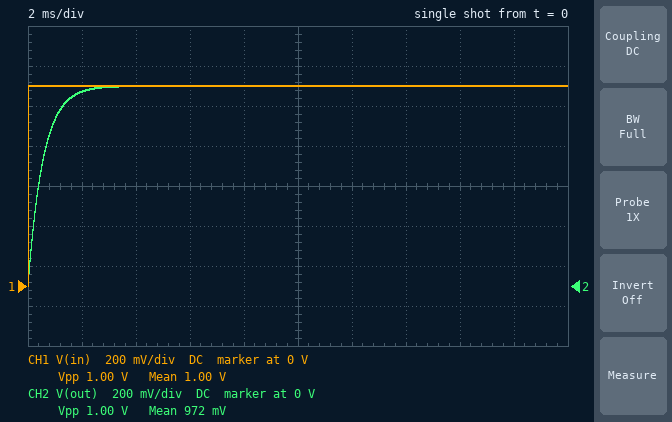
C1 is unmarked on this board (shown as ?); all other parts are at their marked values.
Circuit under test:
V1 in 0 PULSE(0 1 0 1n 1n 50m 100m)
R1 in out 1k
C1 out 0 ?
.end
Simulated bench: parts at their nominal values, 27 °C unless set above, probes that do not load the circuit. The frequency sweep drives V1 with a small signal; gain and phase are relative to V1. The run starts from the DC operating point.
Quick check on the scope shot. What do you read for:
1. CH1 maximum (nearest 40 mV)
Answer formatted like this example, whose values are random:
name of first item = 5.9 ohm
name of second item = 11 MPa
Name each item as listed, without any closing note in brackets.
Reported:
CH1 maximum = 1.00 V
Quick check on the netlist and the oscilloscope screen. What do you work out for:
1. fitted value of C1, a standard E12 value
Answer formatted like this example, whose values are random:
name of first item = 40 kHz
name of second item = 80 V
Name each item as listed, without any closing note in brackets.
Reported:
fitted value of C1, a standard E12 value = 560 nF
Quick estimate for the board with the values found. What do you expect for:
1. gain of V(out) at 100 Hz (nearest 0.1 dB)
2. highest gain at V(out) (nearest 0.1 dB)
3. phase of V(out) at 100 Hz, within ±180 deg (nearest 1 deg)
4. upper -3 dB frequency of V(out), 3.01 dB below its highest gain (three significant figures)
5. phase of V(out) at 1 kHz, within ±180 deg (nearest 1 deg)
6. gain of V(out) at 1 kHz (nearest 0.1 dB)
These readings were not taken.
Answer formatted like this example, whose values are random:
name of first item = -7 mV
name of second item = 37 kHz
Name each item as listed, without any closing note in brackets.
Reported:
gain of V(out) at 100 Hz = -0.5 dB
highest gain at V(out) = 0 dB
phase of V(out) at 100 Hz, within ±180 deg = -19 deg
upper -3 dB frequency of V(out), 3.01 dB below its highest gain = 284 Hz
phase of V(out) at 1 kHz, within ±180 deg = -74 deg
gain of V(out) at 1 kHz = -11.3 dB
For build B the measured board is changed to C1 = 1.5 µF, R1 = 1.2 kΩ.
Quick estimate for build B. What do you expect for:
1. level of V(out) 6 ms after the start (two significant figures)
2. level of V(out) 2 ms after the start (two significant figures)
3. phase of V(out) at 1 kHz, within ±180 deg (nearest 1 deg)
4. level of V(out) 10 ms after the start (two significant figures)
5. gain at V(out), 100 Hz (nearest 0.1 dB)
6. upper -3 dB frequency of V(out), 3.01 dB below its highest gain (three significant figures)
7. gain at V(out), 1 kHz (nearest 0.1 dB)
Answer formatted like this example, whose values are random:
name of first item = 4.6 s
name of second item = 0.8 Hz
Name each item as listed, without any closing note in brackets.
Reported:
level of V(out) 6 ms after the start = 960 mV
level of V(out) 2 ms after the start = 670 mV
phase of V(out) at 1 kHz, within ±180 deg = -85 deg
level of V(out) 10 ms after the start = 1.0 V
gain at V(out), 100 Hz = -3.6 dB
upper -3 dB frequency of V(out), 3.01 dB below its highest gain = 88.4 Hz
gain at V(out), 1 kHz = -21.1 dB
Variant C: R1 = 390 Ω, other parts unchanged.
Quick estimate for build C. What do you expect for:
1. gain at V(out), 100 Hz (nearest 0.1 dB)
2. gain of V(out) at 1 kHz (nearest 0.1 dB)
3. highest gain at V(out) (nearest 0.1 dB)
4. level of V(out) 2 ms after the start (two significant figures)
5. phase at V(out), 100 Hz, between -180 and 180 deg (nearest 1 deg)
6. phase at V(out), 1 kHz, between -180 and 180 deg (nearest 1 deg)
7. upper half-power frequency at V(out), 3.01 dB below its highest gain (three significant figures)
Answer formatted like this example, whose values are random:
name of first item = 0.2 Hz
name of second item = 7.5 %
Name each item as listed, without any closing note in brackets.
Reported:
gain at V(out), 100 Hz = -0.1 dB
gain of V(out) at 1 kHz = -4.6 dB
highest gain at V(out) = 0 dB
level of V(out) 2 ms after the start = 1.0 V
phase at V(out), 100 Hz, between -180 and 180 deg = -8 deg
phase at V(out), 1 kHz, between -180 and 180 deg = -54 deg
upper half-power frequency at V(out), 3.01 dB below its highest gain = 729 Hz
